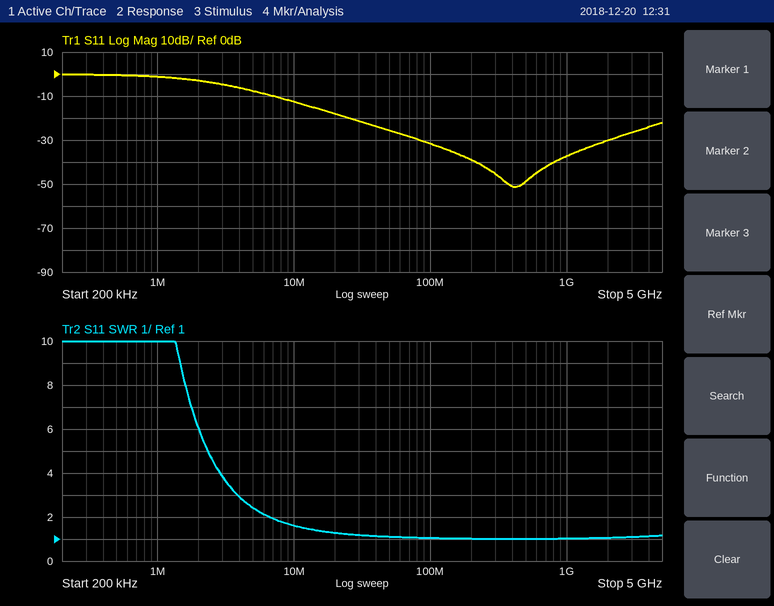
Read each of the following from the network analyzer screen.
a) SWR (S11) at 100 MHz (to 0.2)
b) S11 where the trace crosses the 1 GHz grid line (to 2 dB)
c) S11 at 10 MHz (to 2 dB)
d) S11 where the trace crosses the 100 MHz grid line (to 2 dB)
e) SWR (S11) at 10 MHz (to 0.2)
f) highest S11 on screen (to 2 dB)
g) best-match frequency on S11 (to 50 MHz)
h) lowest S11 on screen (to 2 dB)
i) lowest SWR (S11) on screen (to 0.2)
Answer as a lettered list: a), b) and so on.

a) 1.0
b) -38 dB
c) -12 dB
d) -32 dB
e) 1.6
f) 0 dB
g) 400 MHz
h) -52 dB
i) 1.0
